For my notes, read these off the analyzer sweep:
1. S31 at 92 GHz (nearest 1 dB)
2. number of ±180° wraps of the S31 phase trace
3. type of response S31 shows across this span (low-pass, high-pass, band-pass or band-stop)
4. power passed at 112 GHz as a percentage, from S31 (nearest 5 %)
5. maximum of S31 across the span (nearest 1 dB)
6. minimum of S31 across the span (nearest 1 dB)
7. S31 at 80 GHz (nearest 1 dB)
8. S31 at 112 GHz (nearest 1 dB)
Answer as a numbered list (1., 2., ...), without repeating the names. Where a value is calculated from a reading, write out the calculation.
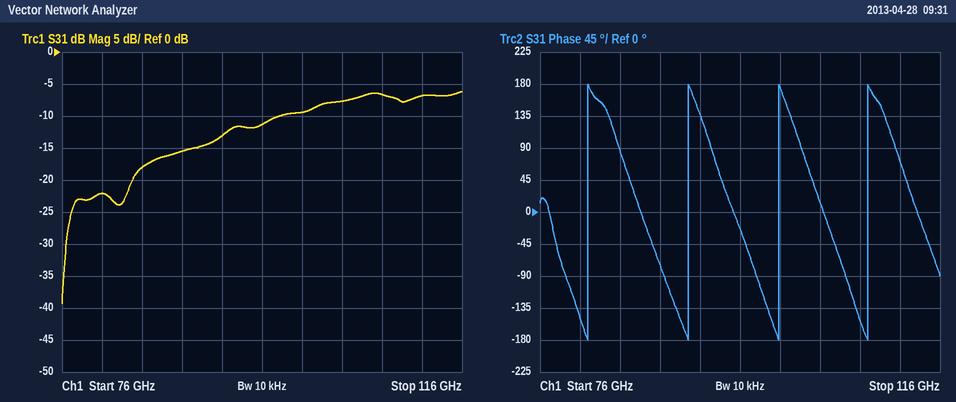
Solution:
1. -13 dB
2. 4
3. high-pass
4. 10^(-7/10) ≈ 20 %
5. -6 dB
6. -39 dB
7. -22 dB
8. -7 dB
